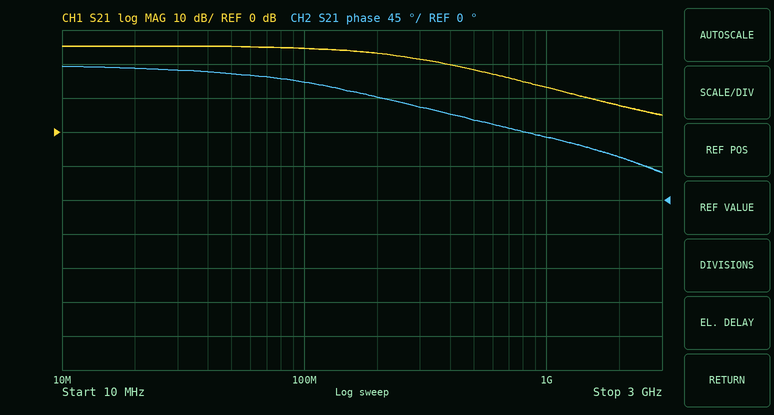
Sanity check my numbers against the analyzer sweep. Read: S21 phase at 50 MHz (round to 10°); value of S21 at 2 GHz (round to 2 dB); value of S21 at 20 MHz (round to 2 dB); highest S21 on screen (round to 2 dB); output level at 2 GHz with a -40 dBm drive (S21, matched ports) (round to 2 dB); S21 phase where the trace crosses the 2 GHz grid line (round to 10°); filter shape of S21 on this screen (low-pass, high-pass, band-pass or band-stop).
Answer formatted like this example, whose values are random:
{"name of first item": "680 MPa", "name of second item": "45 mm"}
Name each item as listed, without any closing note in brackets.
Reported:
{"S21 phase at 50 MHz": "170°", "value of S21 at 2 GHz": "8 dB", "value of S21 at 20 MHz": "26 dB", "highest S21 on screen": "26 dB", "output level at 2 GHz with a -40 dBm drive (S21, matched ports)": "-32 dBm", "S21 phase where the trace crosses the 2 GHz grid line": "60°", "filter shape of S21 on this screen": "low-pass"}
